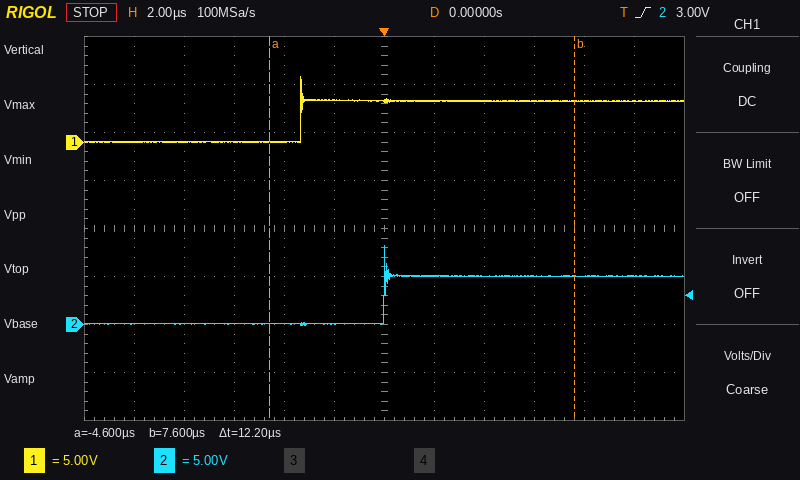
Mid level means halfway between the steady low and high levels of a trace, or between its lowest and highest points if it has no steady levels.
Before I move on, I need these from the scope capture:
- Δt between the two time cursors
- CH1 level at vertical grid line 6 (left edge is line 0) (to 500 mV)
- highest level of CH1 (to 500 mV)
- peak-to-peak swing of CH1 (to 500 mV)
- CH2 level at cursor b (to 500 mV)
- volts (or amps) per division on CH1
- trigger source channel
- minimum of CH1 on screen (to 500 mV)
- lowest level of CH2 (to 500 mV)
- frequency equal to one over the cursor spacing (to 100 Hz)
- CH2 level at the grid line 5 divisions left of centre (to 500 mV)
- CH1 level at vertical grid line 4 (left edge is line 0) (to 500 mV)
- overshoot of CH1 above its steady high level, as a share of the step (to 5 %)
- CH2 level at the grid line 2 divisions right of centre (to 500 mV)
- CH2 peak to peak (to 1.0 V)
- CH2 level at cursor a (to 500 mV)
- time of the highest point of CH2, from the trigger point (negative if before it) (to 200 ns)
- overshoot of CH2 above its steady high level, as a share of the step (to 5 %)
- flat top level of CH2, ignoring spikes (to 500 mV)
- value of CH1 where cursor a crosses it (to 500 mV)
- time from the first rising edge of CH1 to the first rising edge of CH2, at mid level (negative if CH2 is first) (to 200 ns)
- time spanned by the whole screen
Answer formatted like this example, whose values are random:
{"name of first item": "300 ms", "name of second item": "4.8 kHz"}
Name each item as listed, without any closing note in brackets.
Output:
{"Δt between the two time cursors": "12.2 µs", "CH1 level at vertical grid line 6 (left edge is line 0)": "4.5 V", "highest level of CH1": "7.0 V", "peak-to-peak swing of CH1": "7.0 V", "CH2 level at cursor b": "5.0 V", "volts (or amps) per division on CH1": "5 V", "trigger source channel": "CH2", "minimum of CH1 on screen": "0.0 V", "lowest level of CH2": "0.0 V", "frequency equal to one over the cursor spacing": "82.0 kHz", "CH2 level at the grid line 5 divisions left of centre": "0.0 V", "CH1 level at vertical grid line 4 (left edge is line 0)": "0.0 V", "overshoot of CH1 above its steady high level, as a share of the step": "60 %", "CH2 level at the grid line 2 divisions right of centre": "5.0 V", "CH2 peak to peak": "8.0 V", "CH2 level at cursor a": "0.0 V", "time of the highest point of CH2, from the trigger point (negative if before it)": "0.0 µs", "overshoot of CH2 above its steady high level, as a share of the step": "65 %", "flat top level of CH2, ignoring spikes": "5.0 V", "value of CH1 where cursor a crosses it": "0.0 V", "time from the first rising edge of CH1 to the first rising edge of CH2, at mid level (negative if CH2 is first)": "+3.4 µs", "time spanned by the whole screen": "24 µs"}
